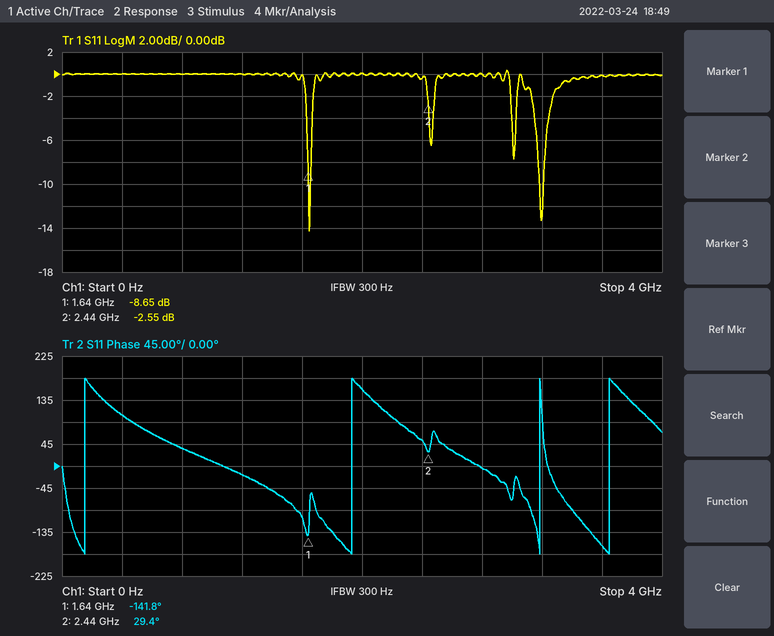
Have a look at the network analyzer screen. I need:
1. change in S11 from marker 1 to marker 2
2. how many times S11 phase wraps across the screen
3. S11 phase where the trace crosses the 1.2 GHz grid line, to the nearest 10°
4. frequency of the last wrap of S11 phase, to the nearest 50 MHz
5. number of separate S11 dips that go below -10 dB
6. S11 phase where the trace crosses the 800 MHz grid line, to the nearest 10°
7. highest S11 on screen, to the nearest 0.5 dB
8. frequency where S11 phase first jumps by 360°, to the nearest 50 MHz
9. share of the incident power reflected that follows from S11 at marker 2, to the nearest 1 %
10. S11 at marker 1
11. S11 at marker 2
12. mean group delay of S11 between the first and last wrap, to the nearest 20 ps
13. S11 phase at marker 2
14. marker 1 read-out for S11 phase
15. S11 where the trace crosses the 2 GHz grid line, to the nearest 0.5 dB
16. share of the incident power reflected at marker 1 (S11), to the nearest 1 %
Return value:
6.10 dB
4
-20°
3.65 GHz
2
40°
0.5 dB
150 MHz
56 %
-8.65 dB
-2.55 dB
860 ps
29.4°
-141.8°
0.0 dB
14 %
